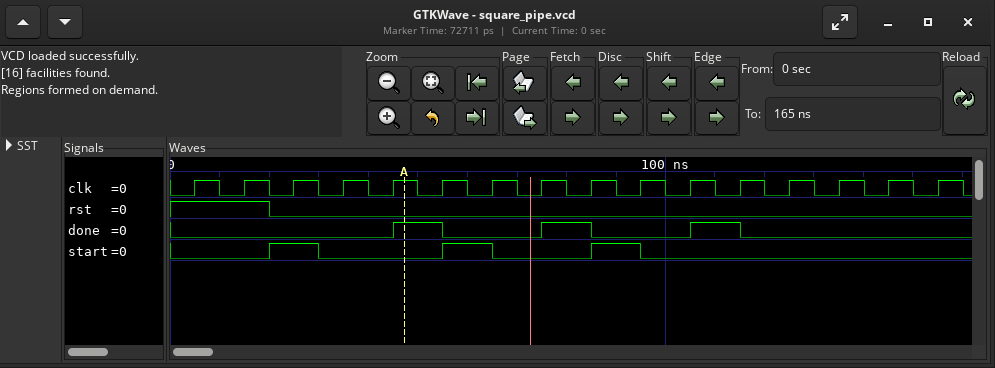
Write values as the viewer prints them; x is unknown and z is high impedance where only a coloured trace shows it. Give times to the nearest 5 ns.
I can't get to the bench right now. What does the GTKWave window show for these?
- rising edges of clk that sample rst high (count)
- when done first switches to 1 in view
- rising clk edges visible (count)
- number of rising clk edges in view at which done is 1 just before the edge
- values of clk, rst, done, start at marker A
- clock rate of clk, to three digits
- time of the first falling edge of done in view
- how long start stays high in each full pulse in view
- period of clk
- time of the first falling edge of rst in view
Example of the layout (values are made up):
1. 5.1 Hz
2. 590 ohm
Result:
1. 2
2. 45 ns
3. 16
4. 3
5. clk=1, rst=0, done=1, start=0
6. 100 MHz
7. 55 ns
8. 10 ns, 10 ns, 10 ns
9. 10 ns
10. 20 ns
